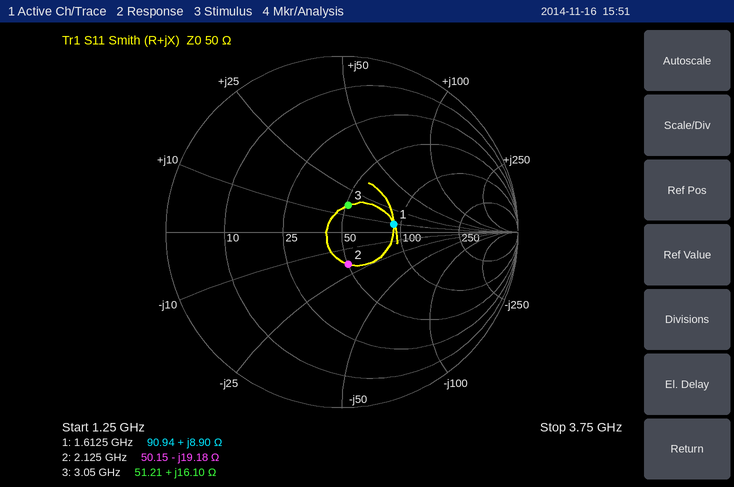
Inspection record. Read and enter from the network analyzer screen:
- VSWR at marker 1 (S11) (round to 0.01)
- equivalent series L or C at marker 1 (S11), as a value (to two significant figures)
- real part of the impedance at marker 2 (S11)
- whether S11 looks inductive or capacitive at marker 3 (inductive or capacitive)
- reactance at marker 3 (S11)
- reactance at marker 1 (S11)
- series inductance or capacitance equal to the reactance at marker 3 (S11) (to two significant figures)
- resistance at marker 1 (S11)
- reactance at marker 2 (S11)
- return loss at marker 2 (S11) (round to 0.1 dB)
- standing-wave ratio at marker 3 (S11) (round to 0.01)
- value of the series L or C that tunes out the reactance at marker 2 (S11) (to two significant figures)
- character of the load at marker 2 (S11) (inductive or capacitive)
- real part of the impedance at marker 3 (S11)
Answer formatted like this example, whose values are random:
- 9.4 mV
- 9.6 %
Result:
- 1.84
- 880 pH
- 50.15 Ω
- inductive
- +16.10 Ω
- +8.90 Ω
- 840 pH
- 90.94 Ω
- -19.18 Ω
- 14.5 dB
- 1.37
- 1.4 nH
- capacitive
- 51.21 Ω
